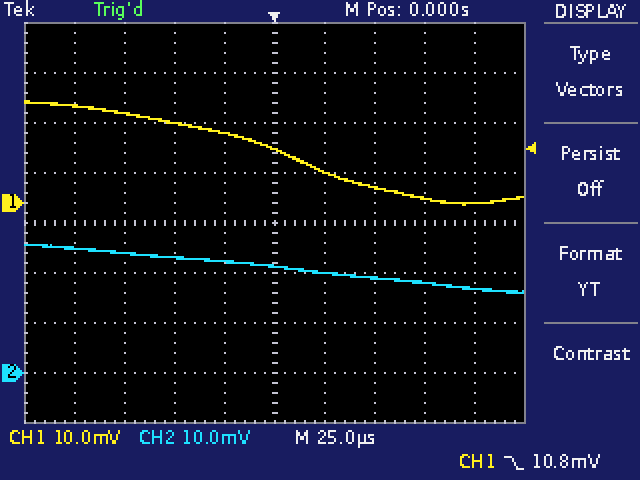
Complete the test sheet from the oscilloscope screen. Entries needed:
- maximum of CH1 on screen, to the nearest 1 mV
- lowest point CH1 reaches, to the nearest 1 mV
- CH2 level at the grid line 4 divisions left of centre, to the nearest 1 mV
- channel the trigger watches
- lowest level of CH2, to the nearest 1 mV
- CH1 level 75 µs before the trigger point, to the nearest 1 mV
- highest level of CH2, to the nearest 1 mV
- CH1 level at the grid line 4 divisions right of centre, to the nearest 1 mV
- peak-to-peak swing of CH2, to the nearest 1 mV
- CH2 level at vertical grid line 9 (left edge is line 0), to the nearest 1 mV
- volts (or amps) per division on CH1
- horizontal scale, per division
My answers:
20 mV
0 mV
25 mV
CH1
16 mV
18 mV
26 mV
0 mV
10 mV
17 mV
10 mV
25 µs
